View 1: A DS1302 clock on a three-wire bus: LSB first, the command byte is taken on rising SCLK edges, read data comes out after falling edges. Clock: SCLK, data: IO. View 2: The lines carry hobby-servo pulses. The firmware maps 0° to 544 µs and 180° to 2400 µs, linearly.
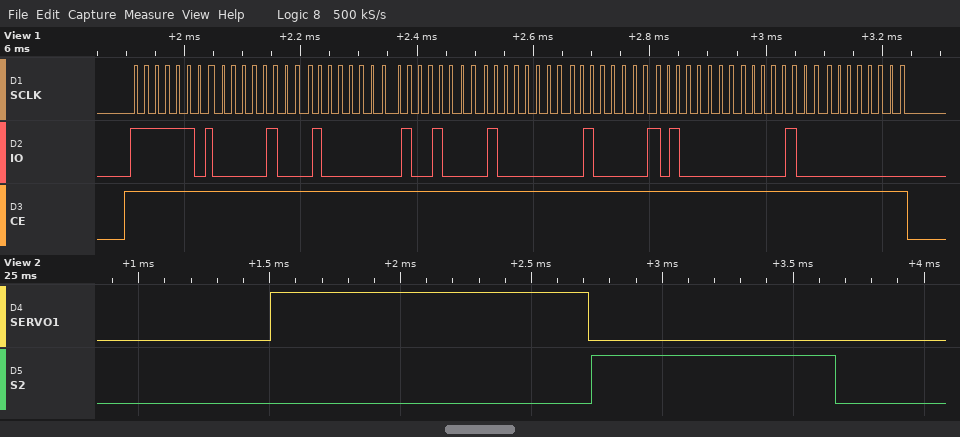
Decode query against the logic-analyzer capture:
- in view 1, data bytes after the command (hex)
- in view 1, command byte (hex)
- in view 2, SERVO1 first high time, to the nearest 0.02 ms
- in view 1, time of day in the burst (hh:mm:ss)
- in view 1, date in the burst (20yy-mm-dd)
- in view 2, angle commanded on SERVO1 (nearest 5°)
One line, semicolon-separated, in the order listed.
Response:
20 02 12 02 04 05 20 00; 0xBF; 1.22 ms; 12:02:20; 2020-04-02; 65°
